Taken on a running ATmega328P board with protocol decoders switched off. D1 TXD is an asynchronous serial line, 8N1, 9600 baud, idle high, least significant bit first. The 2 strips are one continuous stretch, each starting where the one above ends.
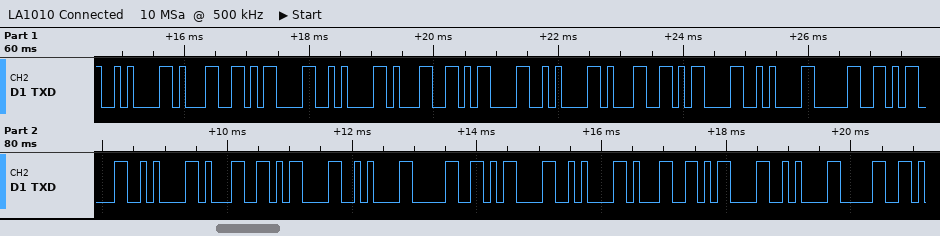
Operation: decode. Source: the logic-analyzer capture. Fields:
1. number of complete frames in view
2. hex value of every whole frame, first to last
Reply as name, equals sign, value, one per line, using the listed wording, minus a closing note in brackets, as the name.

number of complete frames in view = 23
hex value of every whole frame, first to last = 0x0A 0x31 0x0D 0x0A 0x31 0x0D 0x0A 0x31 0x0D 0x0A 0x30 0x0D 0x0A 0x31 0x0D 0x0A 0x30 0x0D 0x0A 0x31 0x0D 0x0A 0x30
